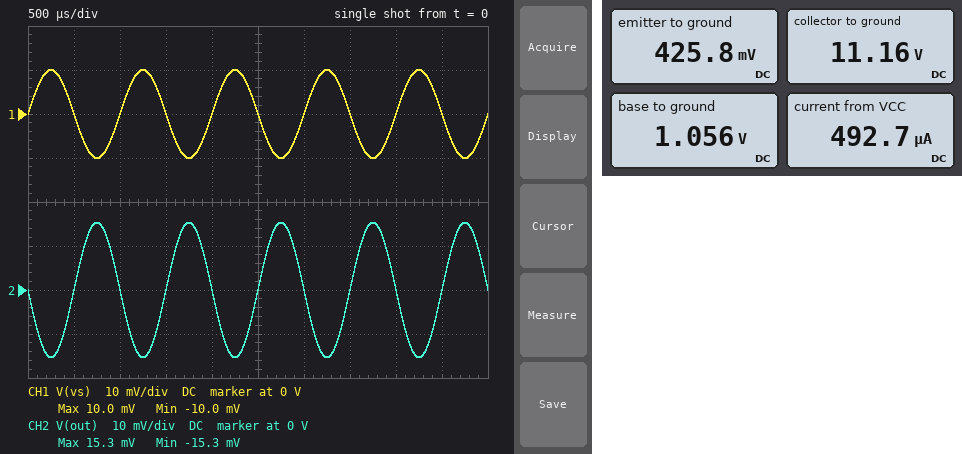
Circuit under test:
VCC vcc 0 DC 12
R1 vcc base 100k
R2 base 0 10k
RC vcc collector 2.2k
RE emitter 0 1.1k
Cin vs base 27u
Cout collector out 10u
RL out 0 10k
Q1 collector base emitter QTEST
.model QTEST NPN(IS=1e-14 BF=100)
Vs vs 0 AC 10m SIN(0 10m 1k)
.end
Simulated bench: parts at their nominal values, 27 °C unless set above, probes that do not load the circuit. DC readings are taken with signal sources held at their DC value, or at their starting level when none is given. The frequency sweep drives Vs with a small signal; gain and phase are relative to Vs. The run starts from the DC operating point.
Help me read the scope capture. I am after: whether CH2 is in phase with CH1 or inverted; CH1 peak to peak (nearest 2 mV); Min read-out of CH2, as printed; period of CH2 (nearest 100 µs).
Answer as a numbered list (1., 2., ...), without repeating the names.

1. inverted
2. 20 mV
3. -15.3 mV
4. 1.0 ms
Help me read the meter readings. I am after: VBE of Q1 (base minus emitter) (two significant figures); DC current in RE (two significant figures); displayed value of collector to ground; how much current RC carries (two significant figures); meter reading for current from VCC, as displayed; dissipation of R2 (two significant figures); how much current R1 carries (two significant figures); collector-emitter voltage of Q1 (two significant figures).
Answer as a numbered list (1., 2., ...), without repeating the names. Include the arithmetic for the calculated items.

1. 1.056 V - 425.8 mV = 630 mV
2. (425.8 mV) / 1.1 kΩ = 390 µA
3. 11.16 V
4. (12 V - 11.16 V) / 2.2 kΩ = 380 µA
5. 492.7 µA
6. (1.056 V)^2 / 10 kΩ = 110 µW
7. (12 V - 1.056 V) / 100 kΩ = 110 µA
8. 11.16 V - 425.8 mV = 11 V
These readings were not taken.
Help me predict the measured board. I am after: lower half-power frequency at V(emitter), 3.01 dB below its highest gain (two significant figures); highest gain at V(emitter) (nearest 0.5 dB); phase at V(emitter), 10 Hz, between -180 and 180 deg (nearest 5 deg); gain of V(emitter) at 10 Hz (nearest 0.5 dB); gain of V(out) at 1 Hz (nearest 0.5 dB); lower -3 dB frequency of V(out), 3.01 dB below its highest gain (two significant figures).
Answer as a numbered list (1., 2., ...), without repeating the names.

1. 700 mHz
2. -0.5 dB
3. 5 deg
4. -0.5 dB
5. -2.5 dB
6. 1.6 Hz
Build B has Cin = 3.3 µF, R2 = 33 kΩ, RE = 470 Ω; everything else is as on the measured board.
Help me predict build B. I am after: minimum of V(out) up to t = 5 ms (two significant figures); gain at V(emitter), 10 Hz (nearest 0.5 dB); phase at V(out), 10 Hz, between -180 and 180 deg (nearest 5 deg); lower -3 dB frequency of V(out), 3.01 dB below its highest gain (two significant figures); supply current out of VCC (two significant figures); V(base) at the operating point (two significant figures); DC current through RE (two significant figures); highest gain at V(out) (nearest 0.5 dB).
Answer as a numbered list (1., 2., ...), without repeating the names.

1. -37 mV
2. -0.5 dB
3. -155 deg
4. 3.4 Hz
5. 3.3 mA
6. 2.2 V
7. 3.2 mA
8. 11.5 dB
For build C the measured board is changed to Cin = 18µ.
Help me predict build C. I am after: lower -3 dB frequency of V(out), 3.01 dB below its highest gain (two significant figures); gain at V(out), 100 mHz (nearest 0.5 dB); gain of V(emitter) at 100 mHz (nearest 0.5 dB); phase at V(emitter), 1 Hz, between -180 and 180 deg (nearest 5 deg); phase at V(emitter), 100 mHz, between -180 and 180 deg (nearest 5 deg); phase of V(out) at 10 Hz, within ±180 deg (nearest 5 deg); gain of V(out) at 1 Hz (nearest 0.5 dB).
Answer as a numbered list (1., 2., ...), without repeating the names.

1. 1.8 Hz
2. -39.0 dB
3. -21.0 dB
4. 45 deg
5. 85 deg
6. -165 deg
7. -4.0 dB
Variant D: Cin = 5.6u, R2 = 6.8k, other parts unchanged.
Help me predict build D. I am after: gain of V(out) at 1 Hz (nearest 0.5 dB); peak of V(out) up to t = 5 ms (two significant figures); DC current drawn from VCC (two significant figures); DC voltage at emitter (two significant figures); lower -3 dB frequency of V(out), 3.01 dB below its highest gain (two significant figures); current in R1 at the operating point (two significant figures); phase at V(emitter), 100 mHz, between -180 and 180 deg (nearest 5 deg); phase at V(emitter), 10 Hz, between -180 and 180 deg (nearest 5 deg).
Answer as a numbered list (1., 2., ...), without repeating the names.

1. -15.0 dB
2. 14 mV
3. 250 µA
4. 150 mV
5. 5.0 Hz
6. 110 µA
7. 90 deg
8. 25 deg
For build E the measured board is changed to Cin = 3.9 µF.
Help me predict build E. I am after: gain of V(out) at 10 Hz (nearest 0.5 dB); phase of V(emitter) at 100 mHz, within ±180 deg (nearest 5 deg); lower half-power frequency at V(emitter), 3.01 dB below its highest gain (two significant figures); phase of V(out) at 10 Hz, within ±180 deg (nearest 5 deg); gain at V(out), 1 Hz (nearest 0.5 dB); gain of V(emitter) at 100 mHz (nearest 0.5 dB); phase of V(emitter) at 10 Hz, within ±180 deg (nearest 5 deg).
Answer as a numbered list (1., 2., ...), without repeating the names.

1. 2.5 dB
2. 90 deg
3. 4.8 Hz
4. -145 deg
5. -14.5 dB
6. -34.0 dB
7. 25 deg
